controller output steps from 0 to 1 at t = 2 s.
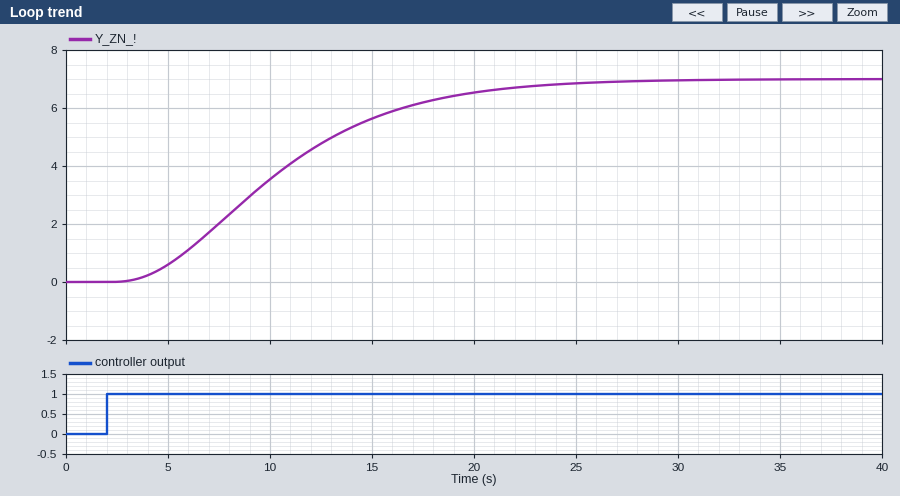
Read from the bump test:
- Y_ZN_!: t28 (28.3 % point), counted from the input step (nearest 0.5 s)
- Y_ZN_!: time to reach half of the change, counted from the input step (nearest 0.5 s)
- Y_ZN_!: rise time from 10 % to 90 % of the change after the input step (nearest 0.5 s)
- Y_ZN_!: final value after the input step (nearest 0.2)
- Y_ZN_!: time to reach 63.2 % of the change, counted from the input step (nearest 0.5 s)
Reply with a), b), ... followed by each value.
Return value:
a) 5.5 s
b) 8.0 s
c) 13.0 s
d) 7.0
e) 9.5 s
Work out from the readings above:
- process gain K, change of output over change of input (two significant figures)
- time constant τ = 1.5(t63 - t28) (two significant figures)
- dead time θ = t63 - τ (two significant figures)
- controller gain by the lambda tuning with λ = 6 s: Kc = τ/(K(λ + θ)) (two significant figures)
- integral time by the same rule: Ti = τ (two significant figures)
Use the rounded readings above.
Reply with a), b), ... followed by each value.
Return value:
a) 7.0
b) 6.0 s
c) 3.5 s
d) 0.090
e) 6.0 s
